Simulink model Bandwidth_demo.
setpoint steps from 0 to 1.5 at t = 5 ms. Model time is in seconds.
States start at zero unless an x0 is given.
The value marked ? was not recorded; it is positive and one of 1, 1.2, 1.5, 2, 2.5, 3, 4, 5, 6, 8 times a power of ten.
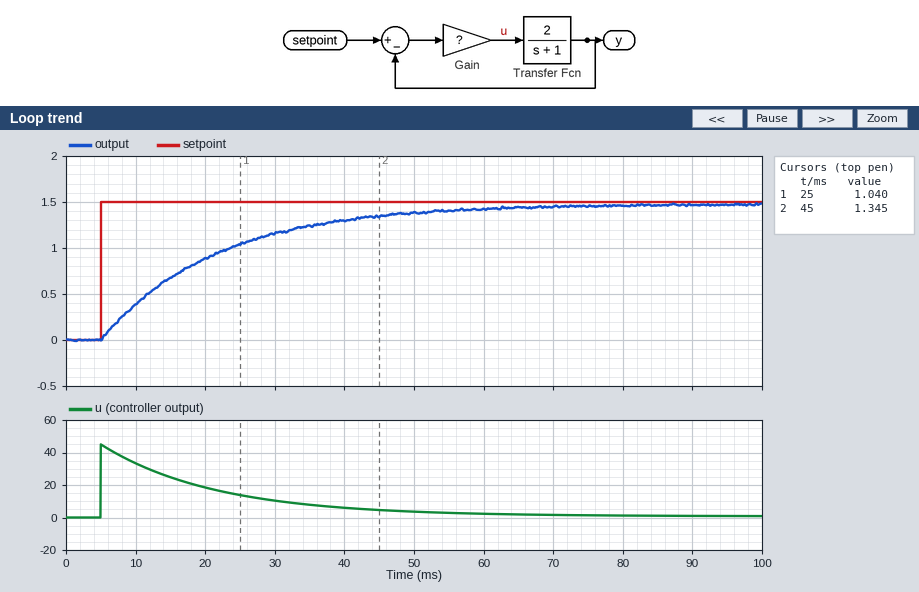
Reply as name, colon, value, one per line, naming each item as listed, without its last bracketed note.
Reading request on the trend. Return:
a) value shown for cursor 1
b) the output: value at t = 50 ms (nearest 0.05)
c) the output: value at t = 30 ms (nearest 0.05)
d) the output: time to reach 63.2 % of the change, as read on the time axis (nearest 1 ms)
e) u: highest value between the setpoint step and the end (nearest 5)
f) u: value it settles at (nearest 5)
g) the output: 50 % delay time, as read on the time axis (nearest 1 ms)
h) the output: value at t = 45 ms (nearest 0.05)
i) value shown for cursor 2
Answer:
value shown for cursor 1: 1.040
the output: value at t = 50 ms: 1.40
the output: value at t = 30 ms: 1.15
the output: time to reach 63.2 % of the change, as read on the time axis: 21 ms
u: highest value between the setpoint step and the end: 45
u: value it settles at: 0
the output: 50 % delay time, as read on the time axis: 16 ms
the output: value at t = 45 ms: 1.35
value shown for cursor 2: 1.345
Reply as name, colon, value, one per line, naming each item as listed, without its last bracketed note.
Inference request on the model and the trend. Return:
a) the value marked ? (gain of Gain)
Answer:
the value marked ?: 30
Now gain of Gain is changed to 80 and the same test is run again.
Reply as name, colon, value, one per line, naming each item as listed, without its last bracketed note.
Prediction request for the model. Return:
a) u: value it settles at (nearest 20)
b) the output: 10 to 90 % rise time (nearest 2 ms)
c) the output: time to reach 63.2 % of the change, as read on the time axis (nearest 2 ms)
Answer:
u: value it settles at: 0
the output: 10 to 90 % rise time: 14 ms
the output: time to reach 63.2 % of the change, as read on the time axis: 12 ms
